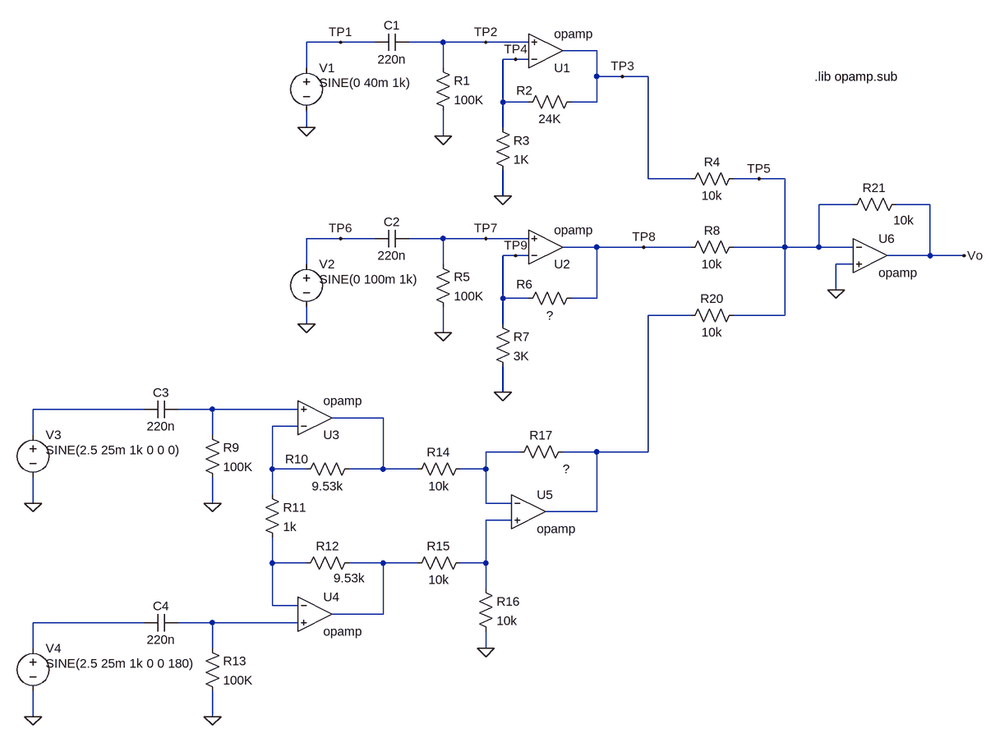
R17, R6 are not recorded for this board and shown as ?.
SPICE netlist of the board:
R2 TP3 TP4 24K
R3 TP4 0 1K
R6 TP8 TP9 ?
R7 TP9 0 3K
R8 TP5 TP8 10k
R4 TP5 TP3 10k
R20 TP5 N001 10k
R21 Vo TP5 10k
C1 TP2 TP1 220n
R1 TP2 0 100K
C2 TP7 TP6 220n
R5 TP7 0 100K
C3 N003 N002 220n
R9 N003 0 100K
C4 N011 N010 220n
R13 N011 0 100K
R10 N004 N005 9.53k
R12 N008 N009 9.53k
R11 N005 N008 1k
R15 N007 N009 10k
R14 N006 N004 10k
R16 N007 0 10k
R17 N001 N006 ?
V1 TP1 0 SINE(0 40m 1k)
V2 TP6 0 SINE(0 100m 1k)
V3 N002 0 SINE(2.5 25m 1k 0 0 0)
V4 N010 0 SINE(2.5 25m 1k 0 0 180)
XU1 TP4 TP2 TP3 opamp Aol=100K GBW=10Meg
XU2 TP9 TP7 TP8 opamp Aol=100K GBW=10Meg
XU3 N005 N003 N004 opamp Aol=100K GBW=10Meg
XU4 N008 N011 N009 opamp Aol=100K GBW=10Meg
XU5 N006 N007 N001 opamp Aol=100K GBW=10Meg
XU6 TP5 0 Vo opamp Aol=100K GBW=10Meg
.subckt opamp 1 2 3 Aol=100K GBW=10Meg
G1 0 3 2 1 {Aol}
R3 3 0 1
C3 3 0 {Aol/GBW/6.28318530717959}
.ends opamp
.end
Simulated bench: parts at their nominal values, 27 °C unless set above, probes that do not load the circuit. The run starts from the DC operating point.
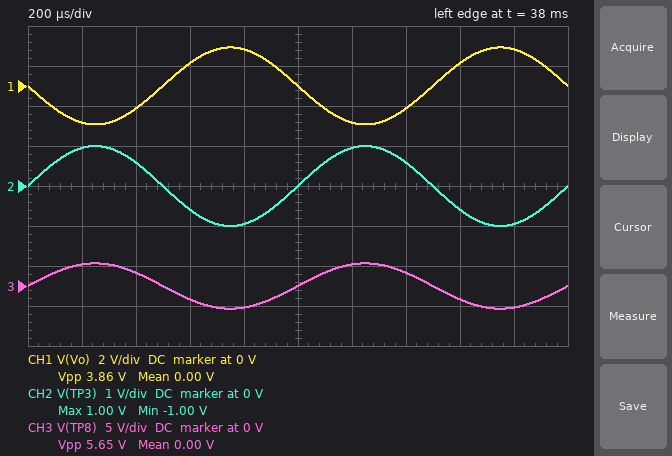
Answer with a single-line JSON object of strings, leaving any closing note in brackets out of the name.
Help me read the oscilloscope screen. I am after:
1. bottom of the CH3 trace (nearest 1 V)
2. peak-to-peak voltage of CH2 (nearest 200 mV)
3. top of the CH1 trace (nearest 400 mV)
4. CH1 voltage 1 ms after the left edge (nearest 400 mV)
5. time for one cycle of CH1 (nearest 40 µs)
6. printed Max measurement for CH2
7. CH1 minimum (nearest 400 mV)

{"bottom of the CH3 trace": "-3 V", "peak-to-peak voltage of CH2": "2.0 V", "top of the CH1 trace": "2.0 V", "CH1 voltage 1 ms after the left edge": "0 V", "time for one cycle of CH1": "1.00 ms", "printed Max measurement for CH2": "1.00 V", "CH1 minimum": "-2.0 V"}
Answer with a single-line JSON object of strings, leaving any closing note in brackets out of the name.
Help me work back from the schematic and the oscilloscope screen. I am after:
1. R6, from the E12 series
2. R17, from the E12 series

{"R6, from the E12 series": "82 kΩ", "R17, from the E12 series": "22 kΩ"}
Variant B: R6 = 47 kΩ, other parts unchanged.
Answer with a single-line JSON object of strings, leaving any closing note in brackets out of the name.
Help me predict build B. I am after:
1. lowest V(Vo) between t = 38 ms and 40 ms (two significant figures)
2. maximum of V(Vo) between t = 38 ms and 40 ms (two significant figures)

{"lowest V(Vo) between t = 38 ms and 40 ms": "-760 mV", "maximum of V(Vo) between t = 38 ms and 40 ms": "760 mV"}
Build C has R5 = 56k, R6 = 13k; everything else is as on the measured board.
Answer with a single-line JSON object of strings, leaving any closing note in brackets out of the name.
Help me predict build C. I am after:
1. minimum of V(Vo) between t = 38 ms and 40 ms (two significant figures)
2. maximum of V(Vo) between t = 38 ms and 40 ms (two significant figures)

{"minimum of V(Vo) between t = 38 ms and 40 ms": "-370 mV", "maximum of V(Vo) between t = 38 ms and 40 ms": "370 mV"}
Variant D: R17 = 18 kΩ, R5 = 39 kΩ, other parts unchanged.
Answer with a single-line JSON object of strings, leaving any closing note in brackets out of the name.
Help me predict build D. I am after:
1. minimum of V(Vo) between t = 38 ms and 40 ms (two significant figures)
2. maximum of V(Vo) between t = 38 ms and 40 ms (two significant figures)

{"minimum of V(Vo) between t = 38 ms and 40 ms": "-2.2 V", "maximum of V(Vo) between t = 38 ms and 40 ms": "2.2 V"}
